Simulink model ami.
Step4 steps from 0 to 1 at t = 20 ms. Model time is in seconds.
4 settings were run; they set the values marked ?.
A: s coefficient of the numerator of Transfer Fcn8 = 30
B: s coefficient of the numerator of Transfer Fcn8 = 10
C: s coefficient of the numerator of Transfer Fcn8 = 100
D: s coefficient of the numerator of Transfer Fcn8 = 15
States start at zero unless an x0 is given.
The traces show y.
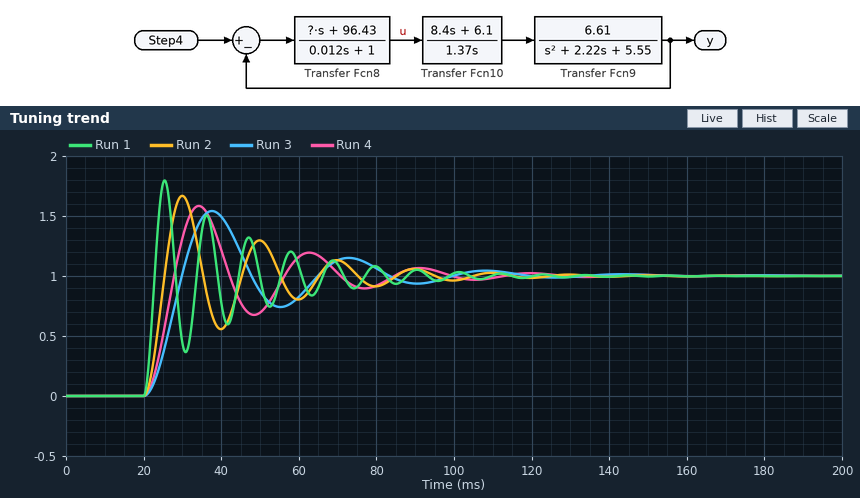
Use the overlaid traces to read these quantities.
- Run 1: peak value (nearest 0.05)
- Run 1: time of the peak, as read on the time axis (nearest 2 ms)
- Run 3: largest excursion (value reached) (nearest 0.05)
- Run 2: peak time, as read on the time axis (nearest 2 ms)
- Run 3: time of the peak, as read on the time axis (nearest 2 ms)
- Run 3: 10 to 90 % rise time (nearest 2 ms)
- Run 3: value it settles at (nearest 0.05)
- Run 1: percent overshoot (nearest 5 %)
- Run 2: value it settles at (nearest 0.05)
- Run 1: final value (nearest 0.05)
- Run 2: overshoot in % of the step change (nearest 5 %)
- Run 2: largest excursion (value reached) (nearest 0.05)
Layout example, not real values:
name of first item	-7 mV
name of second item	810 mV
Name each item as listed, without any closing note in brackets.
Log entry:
Run 1: peak value	1.80
Run 1: time of the peak, as read on the time axis	26 ms
Run 3: largest excursion (value reached)	1.55
Run 2: peak time, as read on the time axis	30 ms
Run 3: time of the peak, as read on the time axis	38 ms
Run 3: 10 to 90 % rise time	6 ms
Run 3: value it settles at	1.00
Run 1: percent overshoot	80 %
Run 2: value it settles at	1.00
Run 1: final value	1.00
Run 2: overshoot in % of the step change	65 %
Run 2: largest excursion (value reached)	1.65
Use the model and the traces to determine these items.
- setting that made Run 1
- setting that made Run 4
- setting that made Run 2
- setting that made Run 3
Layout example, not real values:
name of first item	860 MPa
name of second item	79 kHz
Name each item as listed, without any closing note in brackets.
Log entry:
setting that made Run 1	C
setting that made Run 4	D
setting that made Run 2	A
setting that made Run 3	B
